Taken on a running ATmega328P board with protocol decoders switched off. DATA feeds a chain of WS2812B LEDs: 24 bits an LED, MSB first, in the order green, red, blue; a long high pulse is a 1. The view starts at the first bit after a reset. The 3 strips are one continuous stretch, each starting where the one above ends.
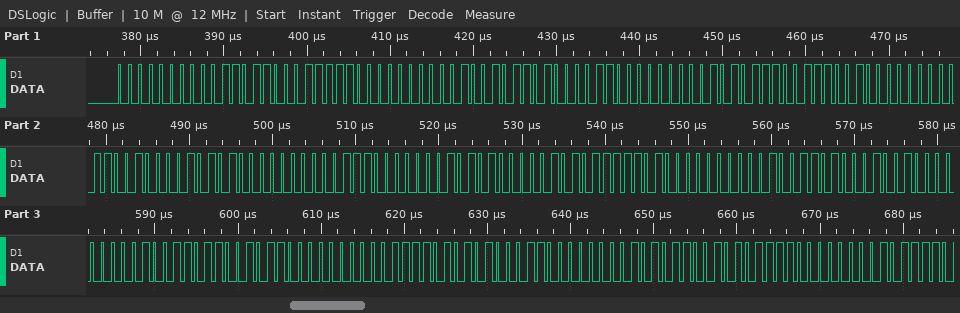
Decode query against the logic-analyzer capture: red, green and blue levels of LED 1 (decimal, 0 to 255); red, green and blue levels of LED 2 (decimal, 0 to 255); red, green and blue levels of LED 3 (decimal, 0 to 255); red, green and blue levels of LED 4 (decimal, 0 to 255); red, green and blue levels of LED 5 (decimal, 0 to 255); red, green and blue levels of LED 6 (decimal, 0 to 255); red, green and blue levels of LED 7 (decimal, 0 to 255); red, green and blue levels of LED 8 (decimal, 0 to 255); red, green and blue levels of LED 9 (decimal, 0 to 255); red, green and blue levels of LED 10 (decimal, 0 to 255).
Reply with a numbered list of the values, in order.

1. 54, 0, 62
2. 75, 0, 67
3. 87, 0, 57
4. 100, 0, 42
5. 112, 0, 21
6. 125, 5, 0
7. 137, 38, 0
8. 150, 77, 0
9. 163, 122, 0
10. 175, 172, 0
